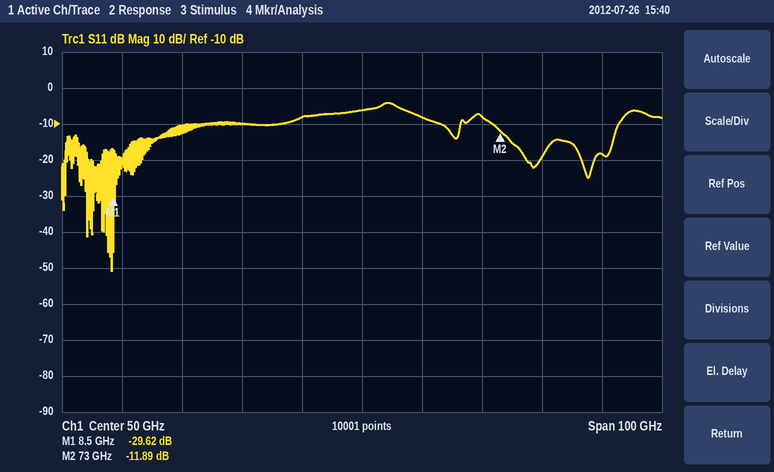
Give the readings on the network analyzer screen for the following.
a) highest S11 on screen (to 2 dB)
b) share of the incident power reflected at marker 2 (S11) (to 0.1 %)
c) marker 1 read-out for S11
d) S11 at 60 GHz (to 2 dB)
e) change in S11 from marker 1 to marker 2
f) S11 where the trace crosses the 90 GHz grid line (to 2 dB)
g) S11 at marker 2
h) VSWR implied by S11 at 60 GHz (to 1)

-4 dB
6.5 %
-29.62 dB
-8 dB
17.73 dB
-18 dB
-11.89 dB
2
